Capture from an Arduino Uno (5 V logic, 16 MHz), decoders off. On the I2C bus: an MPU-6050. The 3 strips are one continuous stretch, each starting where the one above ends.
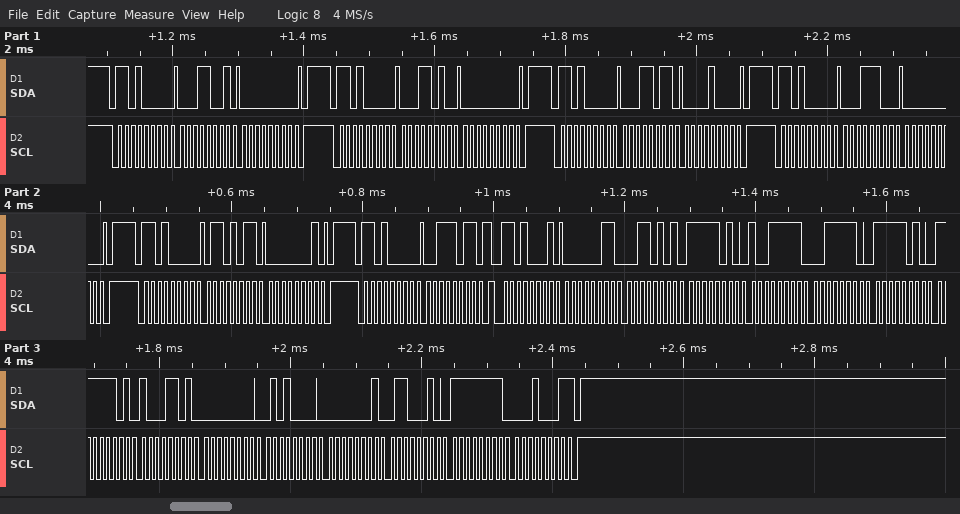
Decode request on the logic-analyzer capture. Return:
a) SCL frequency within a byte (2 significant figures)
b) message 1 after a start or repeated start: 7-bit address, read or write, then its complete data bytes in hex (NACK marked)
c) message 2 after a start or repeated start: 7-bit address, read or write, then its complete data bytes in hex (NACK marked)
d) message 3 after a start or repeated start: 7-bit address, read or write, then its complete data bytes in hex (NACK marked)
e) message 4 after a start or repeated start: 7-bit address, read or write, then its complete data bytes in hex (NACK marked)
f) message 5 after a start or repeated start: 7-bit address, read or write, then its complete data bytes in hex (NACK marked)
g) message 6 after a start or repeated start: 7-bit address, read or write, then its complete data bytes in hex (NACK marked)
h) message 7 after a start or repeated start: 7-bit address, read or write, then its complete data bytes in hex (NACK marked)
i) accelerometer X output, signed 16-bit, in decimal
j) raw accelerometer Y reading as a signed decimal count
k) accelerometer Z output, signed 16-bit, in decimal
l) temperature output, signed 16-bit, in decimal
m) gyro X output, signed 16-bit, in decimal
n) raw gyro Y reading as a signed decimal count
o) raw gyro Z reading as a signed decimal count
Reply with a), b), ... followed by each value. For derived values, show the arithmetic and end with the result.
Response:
a) 100 kHz
b) 0x68 write: 19 00
c) 0x68 write: 1A 00
d) 0x68 write: 1B 08
e) 0x68 write: 1C 00
f) 0x68 write: 6B 01
g) 0x68 write: 3B
h) 0x68 read: 03 35 FA 9F 3E FA FD 8D 00 50 01 62 FF 11 NACK
i) 0x0335 = 821
j) 0xFA9F = -1377
k) 0x3EFA = 16122
l) 0xFD8D = -627
m) 0x0050 = 80
n) 0x0162 = 354
o) 0xFF11 = -239
